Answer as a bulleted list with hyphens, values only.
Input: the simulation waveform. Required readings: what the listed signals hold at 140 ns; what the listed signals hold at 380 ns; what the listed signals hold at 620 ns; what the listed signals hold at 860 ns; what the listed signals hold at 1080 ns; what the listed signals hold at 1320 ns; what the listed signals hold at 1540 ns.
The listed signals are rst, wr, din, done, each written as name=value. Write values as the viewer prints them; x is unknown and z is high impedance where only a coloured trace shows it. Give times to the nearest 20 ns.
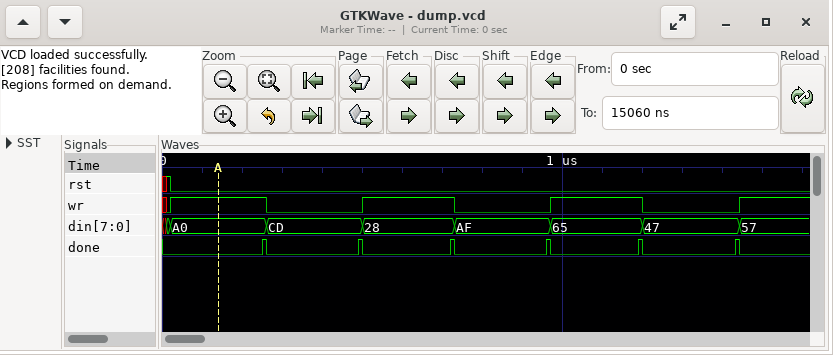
- rst=0, wr=1, din=A0, done=0
- rst=0, wr=0, din=CD, done=0
- rst=0, wr=1, din=28, done=0
- rst=0, wr=0, din=AF, done=0
- rst=0, wr=1, din=65, done=0
- rst=0, wr=0, din=47, done=0
- rst=0, wr=1, din=57, done=0
